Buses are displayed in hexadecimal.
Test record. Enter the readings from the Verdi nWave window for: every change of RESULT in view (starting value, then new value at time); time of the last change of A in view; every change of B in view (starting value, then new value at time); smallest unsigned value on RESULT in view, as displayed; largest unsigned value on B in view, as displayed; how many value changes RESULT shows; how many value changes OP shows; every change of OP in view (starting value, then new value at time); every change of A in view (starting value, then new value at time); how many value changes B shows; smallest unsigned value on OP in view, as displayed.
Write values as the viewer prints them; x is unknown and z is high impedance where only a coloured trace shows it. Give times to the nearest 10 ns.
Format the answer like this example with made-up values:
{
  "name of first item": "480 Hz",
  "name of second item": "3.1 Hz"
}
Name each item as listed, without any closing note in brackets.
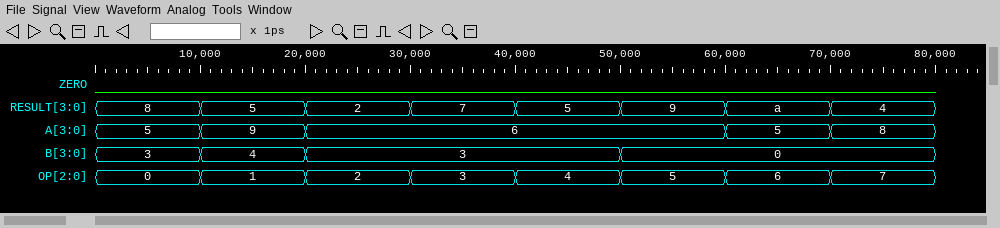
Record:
{
  "every change of RESULT in view": "8, 5 at 10 ns, 2 at 20 ns, 7 at 30 ns, 5 at 40 ns, 9 at 50 ns, a at 60 ns, 4 at 70 ns",
  "time of the last change of A in view": "70 ns",
  "every change of B in view": "3, 4 at 10 ns, 3 at 20 ns, 0 at 50 ns",
  "smallest unsigned value on RESULT in view, as displayed": "2",
  "largest unsigned value on B in view, as displayed": "4",
  "how many value changes RESULT shows": "7",
  "how many value changes OP shows": "7",
  "every change of OP in view": "0, 1 at 10 ns, 2 at 20 ns, 3 at 30 ns, 4 at 40 ns, 5 at 50 ns, 6 at 60 ns, 7 at 70 ns",
  "every change of A in view": "5, 9 at 10 ns, 6 at 20 ns, 5 at 60 ns, 8 at 70 ns",
  "how many value changes B shows": "3",
  "smallest unsigned value on OP in view, as displayed": "0"
}
